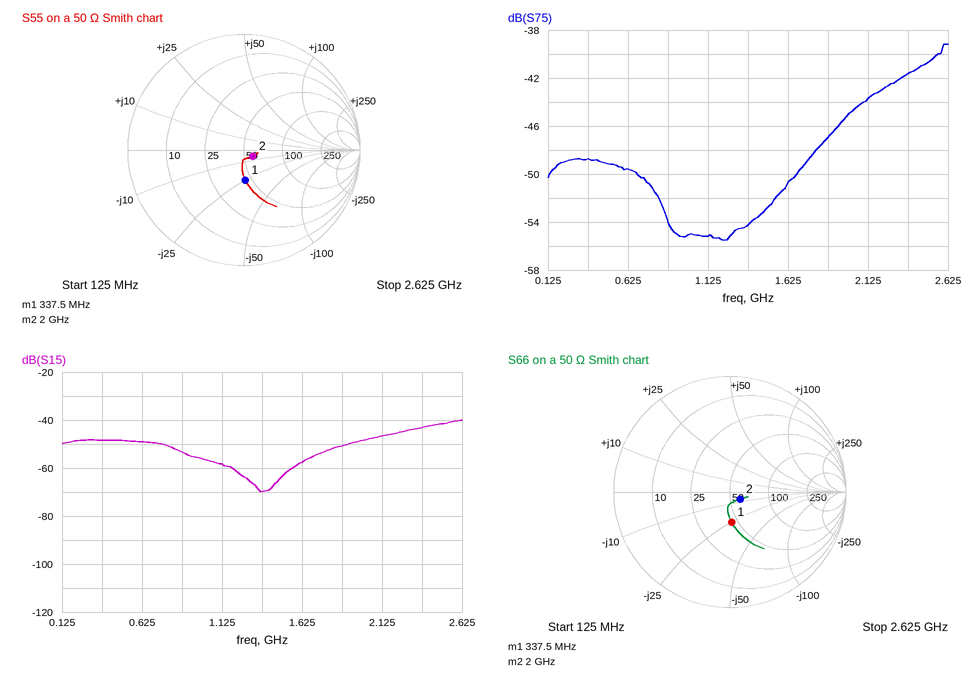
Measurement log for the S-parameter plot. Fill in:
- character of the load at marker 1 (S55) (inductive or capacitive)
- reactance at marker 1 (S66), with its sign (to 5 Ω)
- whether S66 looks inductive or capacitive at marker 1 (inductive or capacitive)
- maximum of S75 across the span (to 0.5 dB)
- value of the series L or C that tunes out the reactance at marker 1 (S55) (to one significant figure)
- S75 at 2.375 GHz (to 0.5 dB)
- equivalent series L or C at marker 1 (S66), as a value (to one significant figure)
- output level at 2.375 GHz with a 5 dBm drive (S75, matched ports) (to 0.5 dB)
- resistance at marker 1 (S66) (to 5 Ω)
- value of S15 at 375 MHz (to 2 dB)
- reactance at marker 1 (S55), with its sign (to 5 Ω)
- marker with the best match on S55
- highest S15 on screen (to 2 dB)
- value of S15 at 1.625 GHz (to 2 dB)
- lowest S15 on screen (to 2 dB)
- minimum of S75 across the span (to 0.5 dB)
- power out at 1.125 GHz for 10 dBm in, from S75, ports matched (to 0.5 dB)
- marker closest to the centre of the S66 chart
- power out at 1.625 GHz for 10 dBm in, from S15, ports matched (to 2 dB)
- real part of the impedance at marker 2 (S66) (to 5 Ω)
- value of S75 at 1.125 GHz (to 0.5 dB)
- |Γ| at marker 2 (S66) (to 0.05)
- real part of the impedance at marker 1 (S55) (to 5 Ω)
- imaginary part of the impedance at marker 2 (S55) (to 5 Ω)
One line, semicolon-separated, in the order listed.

capacitive; -25 Ω; capacitive; -39.0 dB; 10 nH; -41.5 dB; 20 pF; -36.5 dBm; 45 Ω; -48 dB; -25 Ω; marker 2; -40 dB; -58 dB; -70 dB; -55.5 dB; -45.0 dBm; marker 2; -48 dBm; 60 Ω; -55.0 dB; 0.10; 45 Ω; -5 Ω
